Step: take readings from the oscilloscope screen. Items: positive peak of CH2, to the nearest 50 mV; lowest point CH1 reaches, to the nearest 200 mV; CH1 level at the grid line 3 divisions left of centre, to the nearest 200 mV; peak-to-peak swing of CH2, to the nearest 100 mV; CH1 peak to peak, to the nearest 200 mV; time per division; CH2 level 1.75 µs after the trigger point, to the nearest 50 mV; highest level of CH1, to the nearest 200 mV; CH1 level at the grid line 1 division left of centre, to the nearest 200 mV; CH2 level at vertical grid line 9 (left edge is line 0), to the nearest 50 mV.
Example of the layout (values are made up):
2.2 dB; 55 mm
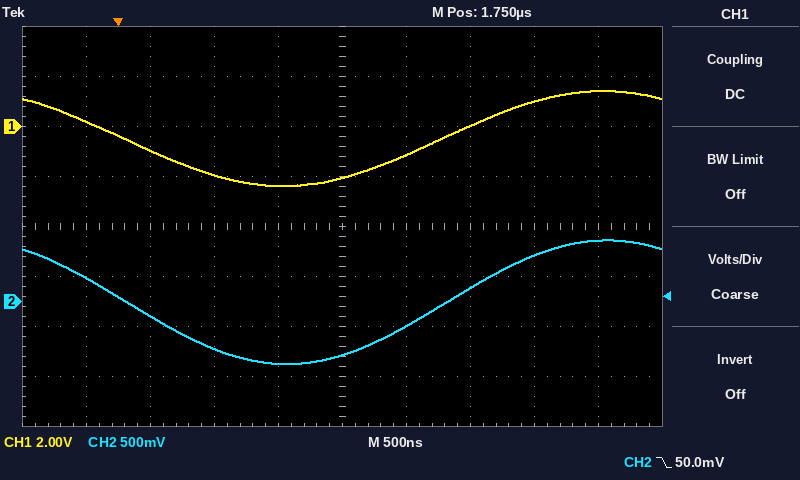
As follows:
600 mV; -2.4 V; -1.0 V; 1.20 V; 3.8 V; 500 ns; -550 mV; 1.4 V; -2.4 V; 600 mV
